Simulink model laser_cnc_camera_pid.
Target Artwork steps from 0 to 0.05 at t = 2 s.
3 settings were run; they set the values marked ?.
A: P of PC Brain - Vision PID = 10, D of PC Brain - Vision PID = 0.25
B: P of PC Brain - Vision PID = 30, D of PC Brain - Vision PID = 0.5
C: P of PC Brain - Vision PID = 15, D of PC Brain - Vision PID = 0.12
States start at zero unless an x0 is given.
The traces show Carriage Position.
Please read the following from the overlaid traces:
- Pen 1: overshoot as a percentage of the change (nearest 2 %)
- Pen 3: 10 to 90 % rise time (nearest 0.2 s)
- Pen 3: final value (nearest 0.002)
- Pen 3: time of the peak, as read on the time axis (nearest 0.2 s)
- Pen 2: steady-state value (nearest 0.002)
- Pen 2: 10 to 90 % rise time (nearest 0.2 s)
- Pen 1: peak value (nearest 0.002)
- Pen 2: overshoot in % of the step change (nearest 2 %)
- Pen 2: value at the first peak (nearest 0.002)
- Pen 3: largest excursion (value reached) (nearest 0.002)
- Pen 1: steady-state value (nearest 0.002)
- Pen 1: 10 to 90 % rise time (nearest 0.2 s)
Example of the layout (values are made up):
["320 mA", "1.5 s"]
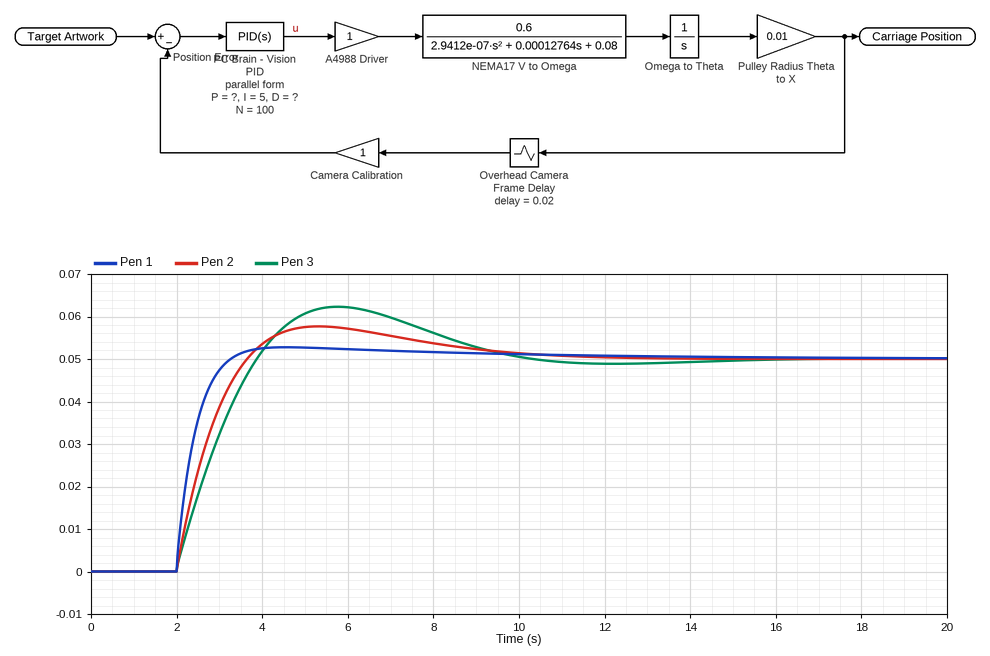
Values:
["6 %", "1.4 s", "0.050", "5.8 s", "0.050", "1.2 s", "0.052", "16 %", "0.058", "0.062", "0.050", "0.8 s"]
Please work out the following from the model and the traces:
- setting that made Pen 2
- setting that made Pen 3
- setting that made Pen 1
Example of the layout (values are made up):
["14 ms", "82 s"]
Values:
["C", "A", "B"]
